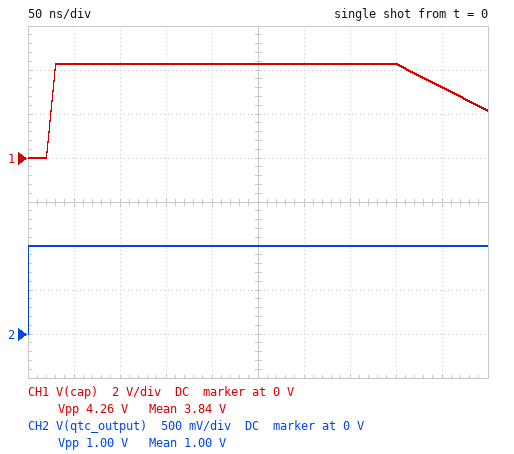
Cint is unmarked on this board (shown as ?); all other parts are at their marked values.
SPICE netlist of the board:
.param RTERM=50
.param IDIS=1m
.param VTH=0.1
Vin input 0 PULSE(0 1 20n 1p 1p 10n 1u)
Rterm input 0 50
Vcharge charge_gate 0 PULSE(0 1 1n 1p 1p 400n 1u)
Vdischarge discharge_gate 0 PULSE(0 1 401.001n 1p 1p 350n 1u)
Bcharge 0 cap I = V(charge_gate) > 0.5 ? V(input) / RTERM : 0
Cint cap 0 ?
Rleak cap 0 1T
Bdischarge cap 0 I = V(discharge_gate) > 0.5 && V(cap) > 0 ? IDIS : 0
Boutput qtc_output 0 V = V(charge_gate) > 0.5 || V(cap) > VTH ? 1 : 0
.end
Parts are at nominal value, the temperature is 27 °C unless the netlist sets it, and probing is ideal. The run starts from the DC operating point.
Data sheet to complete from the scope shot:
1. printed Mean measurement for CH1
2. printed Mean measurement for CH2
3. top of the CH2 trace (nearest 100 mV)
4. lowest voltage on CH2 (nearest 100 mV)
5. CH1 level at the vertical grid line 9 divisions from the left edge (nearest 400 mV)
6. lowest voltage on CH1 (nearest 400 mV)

3.84 V
1.00 V
1.0 V
0 V
3.2 V
0 V
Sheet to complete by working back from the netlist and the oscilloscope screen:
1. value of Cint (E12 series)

47 pF
